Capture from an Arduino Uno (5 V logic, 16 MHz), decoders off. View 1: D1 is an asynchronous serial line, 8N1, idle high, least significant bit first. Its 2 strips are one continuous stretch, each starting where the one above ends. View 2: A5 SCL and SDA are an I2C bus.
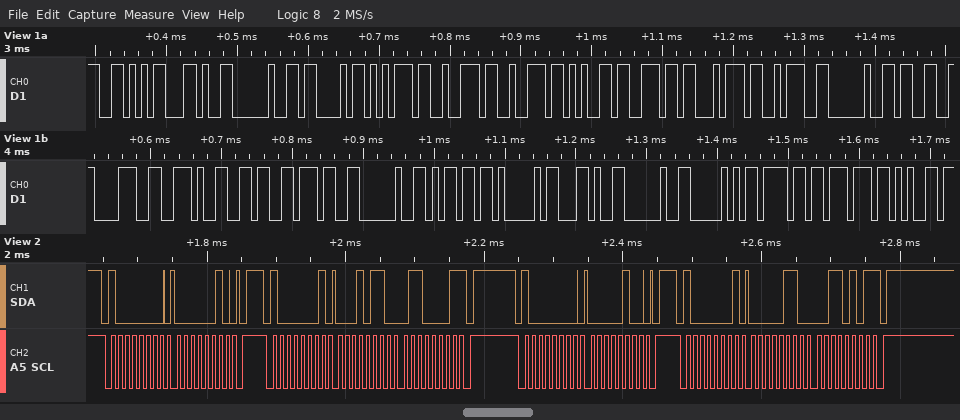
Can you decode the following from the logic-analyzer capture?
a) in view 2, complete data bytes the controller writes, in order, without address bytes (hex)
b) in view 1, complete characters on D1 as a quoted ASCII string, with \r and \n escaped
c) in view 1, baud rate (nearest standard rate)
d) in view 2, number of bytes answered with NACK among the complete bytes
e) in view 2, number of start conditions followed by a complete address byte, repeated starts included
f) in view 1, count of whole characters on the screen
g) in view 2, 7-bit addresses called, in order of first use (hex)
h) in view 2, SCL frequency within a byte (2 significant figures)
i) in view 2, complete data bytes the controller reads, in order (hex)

02 04
"V, Current: 38.67 mA, Powe"
115200 baud
2
4
26
0x40
100 kHz
16 61 06 35
